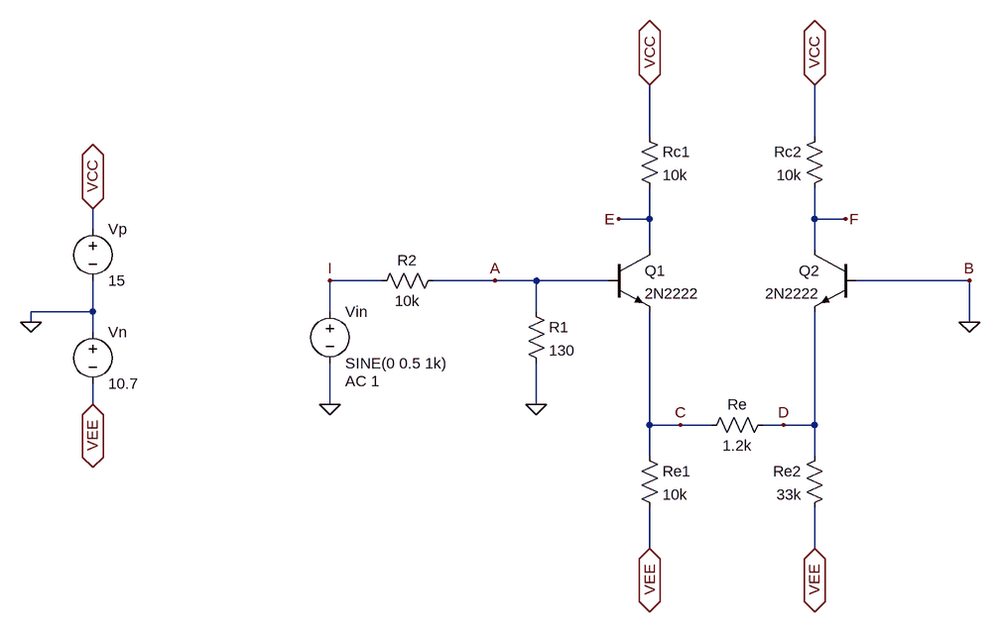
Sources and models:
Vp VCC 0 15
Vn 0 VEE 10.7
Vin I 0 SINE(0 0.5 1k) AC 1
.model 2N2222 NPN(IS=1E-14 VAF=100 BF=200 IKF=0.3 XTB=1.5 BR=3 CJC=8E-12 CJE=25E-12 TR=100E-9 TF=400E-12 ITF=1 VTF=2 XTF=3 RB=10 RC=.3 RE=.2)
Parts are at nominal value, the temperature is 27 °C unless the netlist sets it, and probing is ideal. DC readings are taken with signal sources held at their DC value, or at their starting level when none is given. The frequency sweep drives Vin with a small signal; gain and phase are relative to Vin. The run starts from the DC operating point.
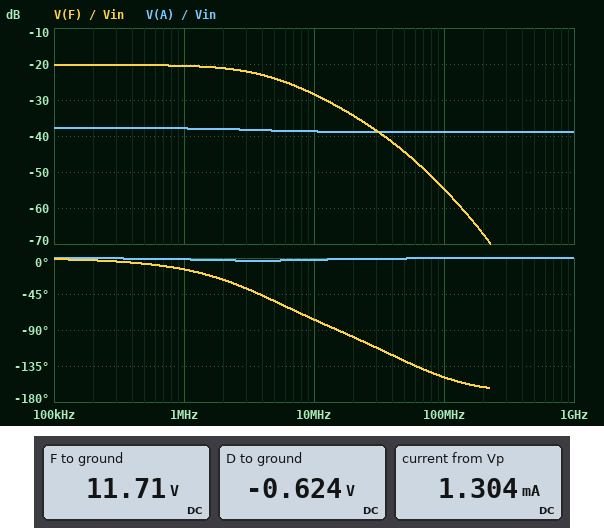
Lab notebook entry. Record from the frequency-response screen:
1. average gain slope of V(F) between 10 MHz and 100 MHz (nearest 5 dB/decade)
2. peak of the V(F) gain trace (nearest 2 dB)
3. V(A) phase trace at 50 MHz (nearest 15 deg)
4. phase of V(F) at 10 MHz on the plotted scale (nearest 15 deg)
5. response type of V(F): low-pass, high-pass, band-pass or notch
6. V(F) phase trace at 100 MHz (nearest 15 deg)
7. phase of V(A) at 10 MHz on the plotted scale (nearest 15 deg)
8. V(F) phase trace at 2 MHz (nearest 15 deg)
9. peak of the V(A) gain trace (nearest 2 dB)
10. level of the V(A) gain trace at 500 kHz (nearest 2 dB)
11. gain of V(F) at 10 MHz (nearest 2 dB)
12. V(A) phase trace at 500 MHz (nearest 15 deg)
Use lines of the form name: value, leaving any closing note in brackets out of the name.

average gain slope of V(F) between 10 MHz and 100 MHz: -25 dB/decade
peak of the V(F) gain trace: -20 dB
V(A) phase trace at 50 MHz: 0 deg
phase of V(F) at 10 MHz on the plotted scale: -75 deg
response type of V(F): low-pass, high-pass, band-pass or notch: low-pass
V(F) phase trace at 100 MHz: -150 deg
phase of V(A) at 10 MHz on the plotted scale: 0 deg
V(F) phase trace at 2 MHz: -30 deg
peak of the V(A) gain trace: -38 dB
level of the V(A) gain trace at 500 kHz: -38 dB
gain of V(F) at 10 MHz: -28 dB
V(A) phase trace at 500 MHz: 0 deg
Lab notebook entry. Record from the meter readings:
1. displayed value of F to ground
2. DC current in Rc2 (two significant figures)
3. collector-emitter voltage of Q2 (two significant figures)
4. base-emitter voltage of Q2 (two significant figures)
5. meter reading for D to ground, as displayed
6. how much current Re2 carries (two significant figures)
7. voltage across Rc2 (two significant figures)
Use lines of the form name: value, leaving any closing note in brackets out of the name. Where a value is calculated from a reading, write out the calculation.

displayed value of F to ground: 11.71 V
DC current in Rc2: (15 V - 11.71 V) / 10 kΩ = 330 µA
collector-emitter voltage of Q2: 11.71 V - (-624 mV) = 12 V
base-emitter voltage of Q2: 0 V - (-624 mV) = 620 mV
meter reading for D to ground, as displayed: -0.624 V
how much current Re2 carries: (-624 mV - (-10.7 V)) / 33 kΩ = 310 µA
voltage across Rc2: 15 V - 11.71 V = 3.3 V
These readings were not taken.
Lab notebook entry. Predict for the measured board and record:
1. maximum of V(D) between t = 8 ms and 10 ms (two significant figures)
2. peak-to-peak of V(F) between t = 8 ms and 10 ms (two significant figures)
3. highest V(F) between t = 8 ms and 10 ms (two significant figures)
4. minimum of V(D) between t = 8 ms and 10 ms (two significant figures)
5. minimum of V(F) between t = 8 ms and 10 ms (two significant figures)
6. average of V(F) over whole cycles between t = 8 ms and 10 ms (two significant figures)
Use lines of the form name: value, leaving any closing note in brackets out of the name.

maximum of V(D) between t = 8 ms and 10 ms: -620 mV
peak-to-peak of V(F) between t = 8 ms and 10 ms: 97 mV
highest V(F) between t = 8 ms and 10 ms: 12 V
minimum of V(D) between t = 8 ms and 10 ms: -620 mV
minimum of V(F) between t = 8 ms and 10 ms: 12 V
average of V(F) over whole cycles between t = 8 ms and 10 ms: 12 V
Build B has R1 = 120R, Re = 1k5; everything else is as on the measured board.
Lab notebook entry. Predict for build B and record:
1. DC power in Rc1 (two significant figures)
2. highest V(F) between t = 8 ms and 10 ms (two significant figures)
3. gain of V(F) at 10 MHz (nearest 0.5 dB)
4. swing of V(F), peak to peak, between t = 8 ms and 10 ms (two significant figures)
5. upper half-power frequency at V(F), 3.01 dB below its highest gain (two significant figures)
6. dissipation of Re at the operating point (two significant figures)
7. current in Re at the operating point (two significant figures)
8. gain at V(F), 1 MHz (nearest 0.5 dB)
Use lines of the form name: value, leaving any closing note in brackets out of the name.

DC power in Rc1: 9.6 mW
highest V(F) between t = 8 ms and 10 ms: 12 V
gain of V(F) at 10 MHz: -30.5 dB
swing of V(F), peak to peak, between t = 8 ms and 10 ms: 73 mV
upper half-power frequency at V(F), 3.01 dB below its highest gain: 4.4 MHz
dissipation of Re at the operating point: 640 nW
current in Re at the operating point: 21 µA
gain at V(F), 1 MHz: -23.0 dB
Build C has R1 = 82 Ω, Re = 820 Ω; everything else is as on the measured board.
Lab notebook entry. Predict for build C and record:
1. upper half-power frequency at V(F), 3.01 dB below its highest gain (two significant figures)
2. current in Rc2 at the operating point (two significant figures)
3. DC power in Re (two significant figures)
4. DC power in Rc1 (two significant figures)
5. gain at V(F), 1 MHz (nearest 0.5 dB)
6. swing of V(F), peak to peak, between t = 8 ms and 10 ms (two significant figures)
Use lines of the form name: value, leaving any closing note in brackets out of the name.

upper half-power frequency at V(F), 3.01 dB below its highest gain: 4.3 MHz
current in Rc2 at the operating point: 340 µA
DC power in Re: 1.0 µW
DC power in Rc1: 9.3 mW
gain at V(F), 1 MHz: -21.5 dB
swing of V(F), peak to peak, between t = 8 ms and 10 ms: 87 mV
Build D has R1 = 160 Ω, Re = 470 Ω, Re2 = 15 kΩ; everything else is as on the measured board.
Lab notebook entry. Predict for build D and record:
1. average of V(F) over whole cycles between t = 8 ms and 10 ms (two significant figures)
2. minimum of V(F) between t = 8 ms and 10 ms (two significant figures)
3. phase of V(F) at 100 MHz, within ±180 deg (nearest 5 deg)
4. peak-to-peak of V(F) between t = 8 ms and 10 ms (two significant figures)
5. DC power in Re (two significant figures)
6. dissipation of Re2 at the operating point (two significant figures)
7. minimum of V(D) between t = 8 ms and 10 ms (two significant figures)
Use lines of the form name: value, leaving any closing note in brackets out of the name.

average of V(F) over whole cycles between t = 8 ms and 10 ms: 8.1 V
minimum of V(F) between t = 8 ms and 10 ms: 8.0 V
phase of V(F) at 100 MHz, within ±180 deg: -135 deg
peak-to-peak of V(F) between t = 8 ms and 10 ms: 290 mV
DC power in Re: 240 nW
dissipation of Re2 at the operating point: 6.7 mW
minimum of V(D) between t = 8 ms and 10 ms: -640 mV
